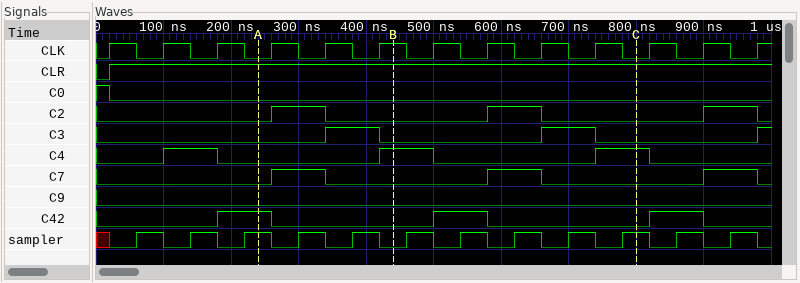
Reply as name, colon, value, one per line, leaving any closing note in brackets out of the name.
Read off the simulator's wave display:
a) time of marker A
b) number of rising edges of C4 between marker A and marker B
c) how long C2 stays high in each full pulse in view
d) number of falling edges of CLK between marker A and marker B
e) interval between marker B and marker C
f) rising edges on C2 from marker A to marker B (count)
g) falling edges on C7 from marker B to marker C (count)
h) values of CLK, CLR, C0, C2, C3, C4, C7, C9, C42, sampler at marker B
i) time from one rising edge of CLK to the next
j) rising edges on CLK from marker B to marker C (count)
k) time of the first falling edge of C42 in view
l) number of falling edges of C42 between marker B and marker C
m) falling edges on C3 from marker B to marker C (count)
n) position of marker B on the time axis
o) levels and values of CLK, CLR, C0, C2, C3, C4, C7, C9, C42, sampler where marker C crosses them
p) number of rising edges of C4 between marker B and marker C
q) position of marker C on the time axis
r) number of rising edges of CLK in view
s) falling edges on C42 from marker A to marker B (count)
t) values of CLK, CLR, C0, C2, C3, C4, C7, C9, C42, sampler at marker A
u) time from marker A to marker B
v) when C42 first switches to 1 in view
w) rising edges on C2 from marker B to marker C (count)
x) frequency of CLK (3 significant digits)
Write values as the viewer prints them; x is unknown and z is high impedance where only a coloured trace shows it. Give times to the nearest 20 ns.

time of marker A: 240 ns
number of rising edges of C4 between marker A and marker B: 1
how long C2 stays high in each full pulse in view: 80 ns, 80 ns, 80 ns
number of falling edges of CLK between marker A and marker B: 2
interval between marker B and marker C: 360 ns
rising edges on C2 from marker A to marker B: 1
falling edges on C7 from marker B to marker C: 1
values of CLK, CLR, C0, C2, C3, C4, C7, C9, C42, sampler at marker B: CLK=1, CLR=1, C0=0, C2=0, C3=0, C4=1, C7=0, C9=0, C42=0, sampler=0
time from one rising edge of CLK to the next: 80 ns
rising edges on CLK from marker B to marker C: 4
time of the first falling edge of C42 in view: 260 ns
number of falling edges of C42 between marker B and marker C: 1
falling edges on C3 from marker B to marker C: 1
position of marker B on the time axis: 440 ns
levels and values of CLK, CLR, C0, C2, C3, C4, C7, C9, C42, sampler where marker C crosses them: CLK=0, CLR=1, C0=0, C2=0, C3=0, C4=1, C7=0, C9=0, C42=0, sampler=1
number of rising edges of C4 between marker B and marker C: 1
position of marker C on the time axis: 800 ns
number of rising edges of CLK in view: 13
falling edges on C42 from marker A to marker B: 1
values of CLK, CLR, C0, C2, C3, C4, C7, C9, C42, sampler at marker A: CLK=0, CLR=1, C0=0, C2=0, C3=0, C4=0, C7=0, C9=0, C42=1, sampler=1
time from marker A to marker B: 200 ns
when C42 first switches to 1 in view: 180 ns
rising edges on C2 from marker B to marker C: 1
frequency of CLK: 12.5 MHz
